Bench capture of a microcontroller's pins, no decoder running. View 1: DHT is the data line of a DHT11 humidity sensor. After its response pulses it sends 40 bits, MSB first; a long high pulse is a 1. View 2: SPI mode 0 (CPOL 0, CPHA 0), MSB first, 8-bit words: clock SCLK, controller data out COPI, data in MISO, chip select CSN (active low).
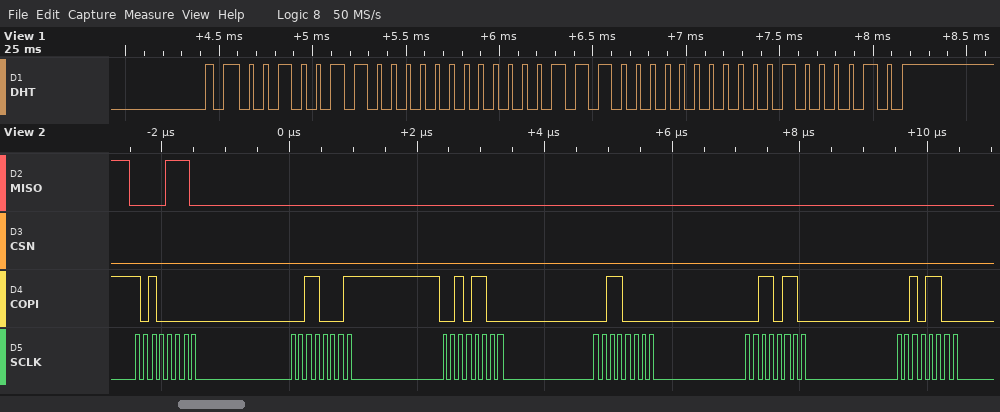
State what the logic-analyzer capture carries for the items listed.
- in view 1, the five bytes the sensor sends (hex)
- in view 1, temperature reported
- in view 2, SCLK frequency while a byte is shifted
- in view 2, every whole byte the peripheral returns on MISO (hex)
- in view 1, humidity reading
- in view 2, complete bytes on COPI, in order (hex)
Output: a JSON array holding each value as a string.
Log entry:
["26 00 1C 00 42", "28.0 °C", "8 MHz", "0E 00 00 00 00 00", "38 %", "A0 31 2C 30 36 2C"]
